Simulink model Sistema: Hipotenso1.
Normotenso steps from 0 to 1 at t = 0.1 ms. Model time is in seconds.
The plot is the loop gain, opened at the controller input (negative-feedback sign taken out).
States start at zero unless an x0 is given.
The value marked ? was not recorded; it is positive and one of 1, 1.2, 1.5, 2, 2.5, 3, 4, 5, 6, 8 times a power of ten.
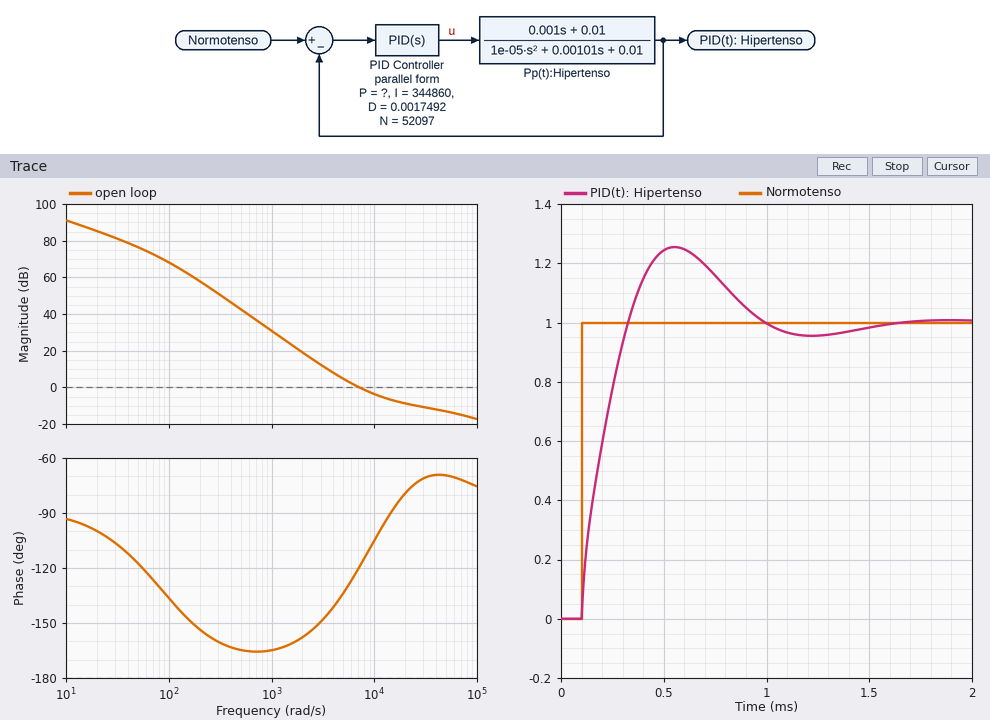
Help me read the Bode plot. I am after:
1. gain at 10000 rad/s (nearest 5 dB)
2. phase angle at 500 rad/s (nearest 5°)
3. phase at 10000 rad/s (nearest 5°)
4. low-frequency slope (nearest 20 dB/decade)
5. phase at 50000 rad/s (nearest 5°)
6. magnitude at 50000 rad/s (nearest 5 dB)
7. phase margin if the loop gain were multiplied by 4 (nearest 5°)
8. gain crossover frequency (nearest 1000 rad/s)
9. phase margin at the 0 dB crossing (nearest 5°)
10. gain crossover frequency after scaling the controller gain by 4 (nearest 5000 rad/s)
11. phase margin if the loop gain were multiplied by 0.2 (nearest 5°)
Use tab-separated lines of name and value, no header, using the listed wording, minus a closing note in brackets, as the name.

gain at 10000 rad/s	-5 dB
phase angle at 500 rad/s	-165°
phase at 10000 rad/s	-105°
low-frequency slope	-20 dB/decade
phase at 50000 rad/s	-70°
magnitude at 50000 rad/s	-15 dB
phase margin if the loop gain were multiplied by 4	110°
gain crossover frequency	7000 rad/s
phase margin at the 0 dB crossing	60°
gain crossover frequency after scaling the controller gain by 4	40000 rad/s
phase margin if the loop gain were multiplied by 0.2	30°
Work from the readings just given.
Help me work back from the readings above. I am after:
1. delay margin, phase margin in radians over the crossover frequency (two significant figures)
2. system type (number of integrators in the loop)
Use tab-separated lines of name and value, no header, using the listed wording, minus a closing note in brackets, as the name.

delay margin, phase margin in radians over the crossover frequency	0.00015 s
system type	1
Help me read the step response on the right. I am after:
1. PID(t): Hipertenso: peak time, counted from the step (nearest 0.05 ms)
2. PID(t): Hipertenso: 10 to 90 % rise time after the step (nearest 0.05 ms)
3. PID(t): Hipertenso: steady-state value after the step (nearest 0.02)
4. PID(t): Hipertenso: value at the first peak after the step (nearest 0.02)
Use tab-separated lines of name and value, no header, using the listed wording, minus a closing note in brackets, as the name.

PID(t): Hipertenso: peak time, counted from the step	0.45 ms
PID(t): Hipertenso: 10 to 90 % rise time after the step	0.20 ms
PID(t): Hipertenso: steady-state value after the step	1.00
PID(t): Hipertenso: value at the first peak after the step	1.26
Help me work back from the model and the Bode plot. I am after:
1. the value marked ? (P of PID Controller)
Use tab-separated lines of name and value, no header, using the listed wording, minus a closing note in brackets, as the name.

the value marked ?	60
